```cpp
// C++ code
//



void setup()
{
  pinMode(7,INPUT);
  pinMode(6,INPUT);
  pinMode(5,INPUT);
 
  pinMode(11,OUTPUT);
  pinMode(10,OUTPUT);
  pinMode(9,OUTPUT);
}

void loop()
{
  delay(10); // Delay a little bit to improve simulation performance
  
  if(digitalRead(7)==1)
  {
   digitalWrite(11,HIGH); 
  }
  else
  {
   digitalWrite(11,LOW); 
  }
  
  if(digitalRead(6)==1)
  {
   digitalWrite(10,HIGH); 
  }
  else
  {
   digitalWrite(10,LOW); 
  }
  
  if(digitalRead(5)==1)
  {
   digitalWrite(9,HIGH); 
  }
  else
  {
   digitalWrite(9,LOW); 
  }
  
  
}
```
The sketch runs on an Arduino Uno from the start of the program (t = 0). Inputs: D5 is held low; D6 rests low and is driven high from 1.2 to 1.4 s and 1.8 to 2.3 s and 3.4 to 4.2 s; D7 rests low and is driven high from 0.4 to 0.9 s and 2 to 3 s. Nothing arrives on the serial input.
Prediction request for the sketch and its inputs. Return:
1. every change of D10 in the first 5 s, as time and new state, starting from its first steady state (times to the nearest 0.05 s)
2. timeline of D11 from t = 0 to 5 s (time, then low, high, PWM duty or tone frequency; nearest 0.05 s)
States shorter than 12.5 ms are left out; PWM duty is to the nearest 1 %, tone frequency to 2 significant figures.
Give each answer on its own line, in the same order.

0 s low; 1.2 s high; 1.4 s low; 1.8 s high; 2.3 s low; 3.4 s high; 4.2 s low
0 s low; 0.4 s high; 0.9 s low; 2 s high; 3 s low
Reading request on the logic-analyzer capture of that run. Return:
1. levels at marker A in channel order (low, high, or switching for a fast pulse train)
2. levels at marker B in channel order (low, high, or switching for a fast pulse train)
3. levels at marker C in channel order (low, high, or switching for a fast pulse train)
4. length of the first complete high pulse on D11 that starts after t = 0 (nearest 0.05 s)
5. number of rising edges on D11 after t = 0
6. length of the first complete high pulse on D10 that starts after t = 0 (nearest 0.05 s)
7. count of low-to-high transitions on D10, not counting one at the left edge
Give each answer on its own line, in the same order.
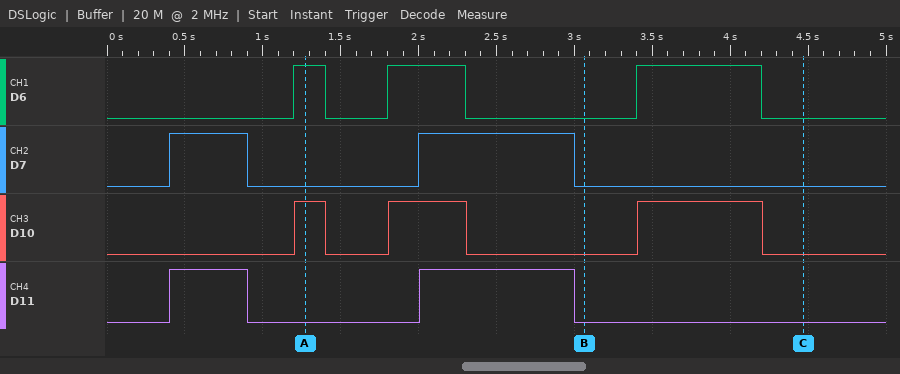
D6 high, D7 low, D10 high, D11 low
D6 low, D7 low, D10 low, D11 low
D6 low, D7 low, D10 low, D11 low
0.50 s
2
0.20 s
3
